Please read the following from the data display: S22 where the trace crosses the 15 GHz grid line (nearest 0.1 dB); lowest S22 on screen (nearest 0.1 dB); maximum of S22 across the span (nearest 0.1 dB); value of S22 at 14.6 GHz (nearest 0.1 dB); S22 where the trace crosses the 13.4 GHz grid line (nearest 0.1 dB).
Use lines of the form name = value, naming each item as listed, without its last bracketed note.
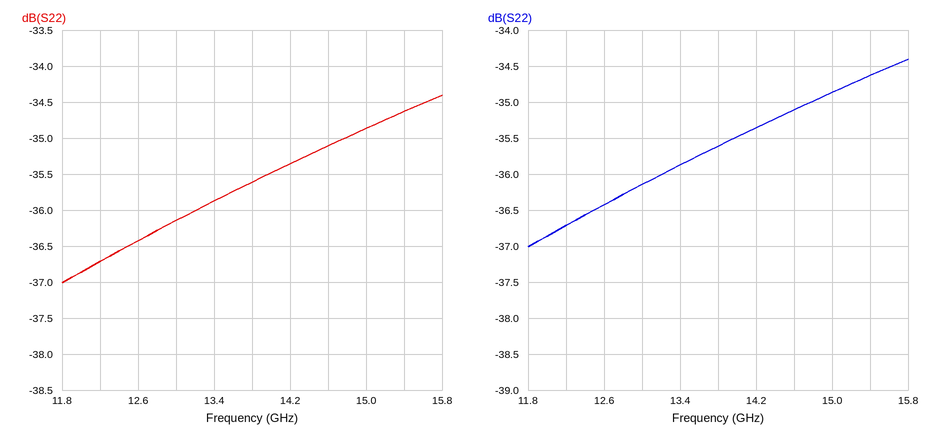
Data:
S22 where the trace crosses the 15 GHz grid line = -34.9 dB
lowest S22 on screen = -37.0 dB
maximum of S22 across the span = -34.4 dB
value of S22 at 14.6 GHz = -35.1 dB
S22 where the trace crosses the 13.4 GHz grid line = -35.9 dB
